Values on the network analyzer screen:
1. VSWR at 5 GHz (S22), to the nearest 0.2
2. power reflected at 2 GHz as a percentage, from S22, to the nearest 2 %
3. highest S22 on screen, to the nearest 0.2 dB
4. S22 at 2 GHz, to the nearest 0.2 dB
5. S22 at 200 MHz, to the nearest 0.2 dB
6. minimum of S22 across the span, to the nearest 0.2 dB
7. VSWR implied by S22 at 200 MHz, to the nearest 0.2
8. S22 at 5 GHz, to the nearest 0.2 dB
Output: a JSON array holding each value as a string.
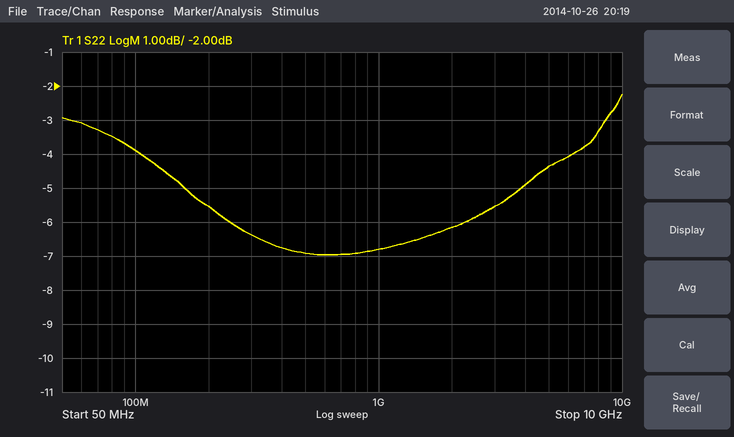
["4.0", "24 %", "-2.2 dB", "-6.2 dB", "-5.6 dB", "-7.0 dB", "3.2", "-4.4 dB"]
